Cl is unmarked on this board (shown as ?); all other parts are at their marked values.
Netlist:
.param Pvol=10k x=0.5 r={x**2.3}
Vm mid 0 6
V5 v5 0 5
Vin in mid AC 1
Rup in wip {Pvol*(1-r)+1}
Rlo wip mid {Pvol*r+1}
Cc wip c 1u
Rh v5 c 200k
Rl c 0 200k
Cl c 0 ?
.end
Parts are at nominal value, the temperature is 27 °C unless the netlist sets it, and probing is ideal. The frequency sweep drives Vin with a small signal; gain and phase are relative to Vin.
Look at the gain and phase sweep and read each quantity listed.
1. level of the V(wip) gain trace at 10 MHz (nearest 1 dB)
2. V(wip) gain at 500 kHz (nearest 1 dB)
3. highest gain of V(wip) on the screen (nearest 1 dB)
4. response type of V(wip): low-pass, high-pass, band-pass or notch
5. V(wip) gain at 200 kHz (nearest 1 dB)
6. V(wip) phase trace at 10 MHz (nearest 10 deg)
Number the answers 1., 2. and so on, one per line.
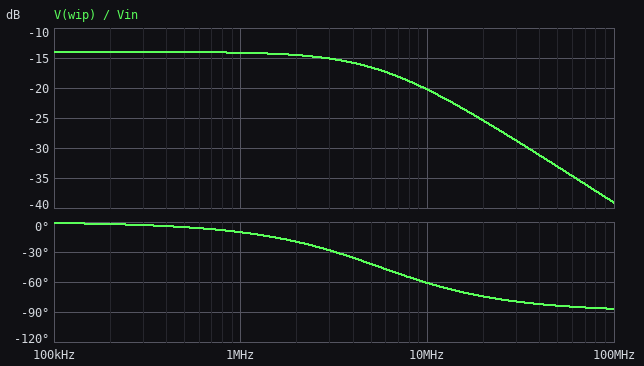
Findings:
1. -20 dB
2. -14 dB
3. -14 dB
4. low-pass
5. -14 dB
6. -60 deg
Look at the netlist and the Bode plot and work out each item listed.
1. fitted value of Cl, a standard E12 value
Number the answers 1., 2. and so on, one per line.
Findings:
1. 18 pF
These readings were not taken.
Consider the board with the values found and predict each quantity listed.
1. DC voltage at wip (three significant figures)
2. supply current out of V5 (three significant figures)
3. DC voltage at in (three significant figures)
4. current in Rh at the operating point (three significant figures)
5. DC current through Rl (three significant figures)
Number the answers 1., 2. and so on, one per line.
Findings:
1. 6.00 V
2. 12.5 µA
3. 6.00 V
4. 12.5 µA
5. 12.5 µA
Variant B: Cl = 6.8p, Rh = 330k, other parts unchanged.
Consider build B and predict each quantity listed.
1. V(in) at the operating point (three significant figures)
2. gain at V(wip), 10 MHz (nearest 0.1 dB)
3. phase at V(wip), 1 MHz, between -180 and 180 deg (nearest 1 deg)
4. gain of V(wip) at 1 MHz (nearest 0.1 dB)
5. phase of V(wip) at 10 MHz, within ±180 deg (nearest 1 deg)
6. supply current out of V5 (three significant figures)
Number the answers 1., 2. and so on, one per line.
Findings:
1. 6.00 V
2. -15.6 dB
3. -4 deg
4. -14.0 dB
5. -34 deg
6. 9.43 µA
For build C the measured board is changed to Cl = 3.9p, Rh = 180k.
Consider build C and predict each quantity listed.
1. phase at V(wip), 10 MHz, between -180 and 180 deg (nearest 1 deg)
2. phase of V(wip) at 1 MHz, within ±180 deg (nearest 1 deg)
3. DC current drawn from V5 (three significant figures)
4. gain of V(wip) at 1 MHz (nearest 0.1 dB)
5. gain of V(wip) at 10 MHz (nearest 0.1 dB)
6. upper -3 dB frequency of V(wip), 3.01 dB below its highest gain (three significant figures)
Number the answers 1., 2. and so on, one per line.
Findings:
1. -21 deg
2. -2 deg
3. 13.2 µA
4. -14.0 dB
5. -14.6 dB
6. 25.6 MHz
